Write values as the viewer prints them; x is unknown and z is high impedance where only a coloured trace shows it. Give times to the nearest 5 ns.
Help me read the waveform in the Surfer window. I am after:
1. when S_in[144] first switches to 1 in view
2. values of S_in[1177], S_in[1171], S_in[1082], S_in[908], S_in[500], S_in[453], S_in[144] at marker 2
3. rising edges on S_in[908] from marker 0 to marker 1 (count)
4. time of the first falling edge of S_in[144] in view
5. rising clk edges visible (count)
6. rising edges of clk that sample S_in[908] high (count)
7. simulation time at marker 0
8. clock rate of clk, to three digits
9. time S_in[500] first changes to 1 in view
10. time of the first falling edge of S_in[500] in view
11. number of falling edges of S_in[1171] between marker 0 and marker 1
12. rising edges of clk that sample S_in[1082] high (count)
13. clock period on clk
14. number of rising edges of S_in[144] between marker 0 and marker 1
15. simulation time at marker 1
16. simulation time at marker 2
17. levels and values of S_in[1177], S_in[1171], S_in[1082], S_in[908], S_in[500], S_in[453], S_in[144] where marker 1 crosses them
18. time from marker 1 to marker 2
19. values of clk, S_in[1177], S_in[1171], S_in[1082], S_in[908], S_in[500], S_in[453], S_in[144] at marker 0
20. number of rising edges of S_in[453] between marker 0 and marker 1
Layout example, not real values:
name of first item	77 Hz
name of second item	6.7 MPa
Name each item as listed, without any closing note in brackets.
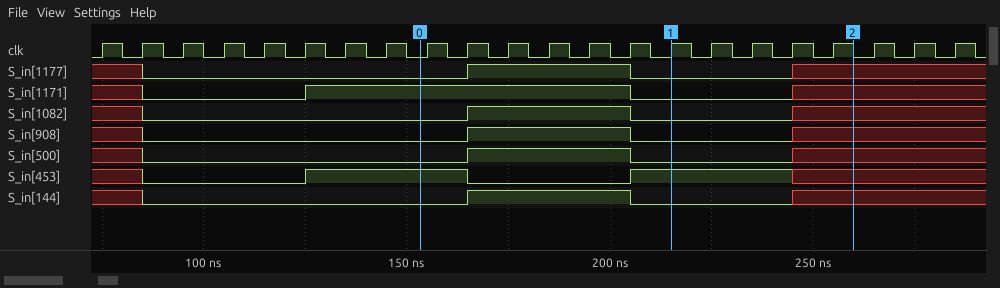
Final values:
when S_in[144] first switches to 1 in view	165 ns
values of S_in[1177], S_in[1171], S_in[1082], S_in[908], S_in[500], S_in[453], S_in[144] at marker 2	S_in[1177]=x, S_in[1171]=x, S_in[1082]=x, S_in[908]=x, S_in[500]=x, S_in[453]=x, S_in[144]=x
rising edges on S_in[908] from marker 0 to marker 1	1
time of the first falling edge of S_in[144] in view	205 ns
rising clk edges visible	22
rising edges of clk that sample S_in[908] high	4
simulation time at marker 0	155 ns
clock rate of clk, to three digits	100 MHz
time S_in[500] first changes to 1 in view	165 ns
time of the first falling edge of S_in[500] in view	205 ns
number of falling edges of S_in[1171] between marker 0 and marker 1	1
rising edges of clk that sample S_in[1082] high	4
clock period on clk	10 ns
number of rising edges of S_in[144] between marker 0 and marker 1	1
simulation time at marker 1	215 ns
simulation time at marker 2	260 ns
levels and values of S_in[1177], S_in[1171], S_in[1082], S_in[908], S_in[500], S_in[453], S_in[144] where marker 1 crosses them	S_in[1177]=0, S_in[1171]=0, S_in[1082]=0, S_in[908]=0, S_in[500]=0, S_in[453]=1, S_in[144]=0
time from marker 1 to marker 2	45 ns
values of clk, S_in[1177], S_in[1171], S_in[1082], S_in[908], S_in[500], S_in[453], S_in[144] at marker 0	clk=0, S_in[1177]=0, S_in[1171]=1, S_in[1082]=0, S_in[908]=0, S_in[500]=0, S_in[453]=1, S_in[144]=0
number of rising edges of S_in[453] between marker 0 and marker 1	1
